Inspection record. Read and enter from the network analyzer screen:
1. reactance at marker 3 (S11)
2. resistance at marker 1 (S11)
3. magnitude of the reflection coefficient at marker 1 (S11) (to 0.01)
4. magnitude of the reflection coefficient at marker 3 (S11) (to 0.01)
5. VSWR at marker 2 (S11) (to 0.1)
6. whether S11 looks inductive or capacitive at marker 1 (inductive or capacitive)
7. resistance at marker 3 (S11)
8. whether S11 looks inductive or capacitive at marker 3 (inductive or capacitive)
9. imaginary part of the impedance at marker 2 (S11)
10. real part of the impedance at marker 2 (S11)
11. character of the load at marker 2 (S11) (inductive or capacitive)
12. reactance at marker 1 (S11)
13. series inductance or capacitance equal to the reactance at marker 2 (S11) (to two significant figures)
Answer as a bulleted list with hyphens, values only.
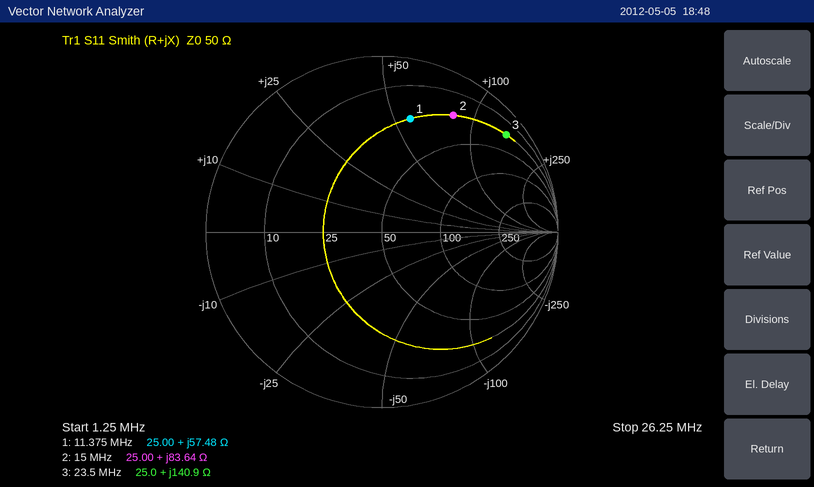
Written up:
- +140.9 Ω
- 25.00 Ω
- 0.66
- 0.90
- 8.0
- inductive
- 25.0 Ω
- inductive
- +83.64 Ω
- 25.00 Ω
- inductive
- +57.48 Ω
- 890 nH
